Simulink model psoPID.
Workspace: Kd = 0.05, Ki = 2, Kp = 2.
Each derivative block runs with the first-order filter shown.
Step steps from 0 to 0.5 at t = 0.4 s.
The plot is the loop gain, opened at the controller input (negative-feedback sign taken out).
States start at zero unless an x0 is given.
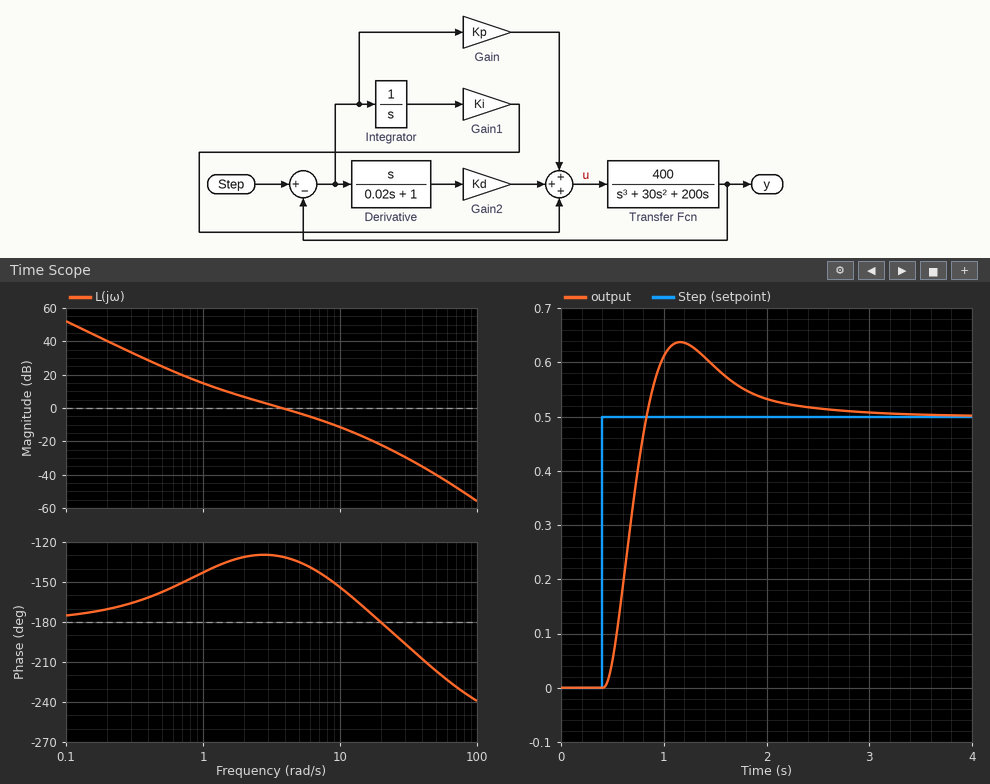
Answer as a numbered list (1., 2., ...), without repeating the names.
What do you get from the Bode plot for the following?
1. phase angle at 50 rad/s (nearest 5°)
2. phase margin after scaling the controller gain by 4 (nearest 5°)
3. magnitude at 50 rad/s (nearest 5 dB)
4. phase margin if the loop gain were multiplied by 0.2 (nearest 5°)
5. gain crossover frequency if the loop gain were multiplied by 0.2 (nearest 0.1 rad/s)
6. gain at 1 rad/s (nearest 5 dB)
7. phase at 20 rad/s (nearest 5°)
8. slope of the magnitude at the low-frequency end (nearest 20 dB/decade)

1. -215°
2. 25°
3. -40 dB
4. 40°
5. 1.1 rad/s
6. 15 dB
7. -180°
8. -40 dB/decade
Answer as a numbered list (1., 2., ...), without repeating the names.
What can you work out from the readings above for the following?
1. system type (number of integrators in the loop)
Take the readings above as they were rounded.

1. 2
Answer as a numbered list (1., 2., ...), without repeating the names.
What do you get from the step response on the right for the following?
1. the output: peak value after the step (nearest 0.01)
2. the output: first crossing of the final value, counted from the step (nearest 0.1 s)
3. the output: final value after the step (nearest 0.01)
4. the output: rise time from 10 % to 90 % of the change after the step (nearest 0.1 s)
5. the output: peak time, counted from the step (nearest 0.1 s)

1. 0.64
2. 0.4 s
3. 0.50
4. 0.3 s
5. 0.8 s
